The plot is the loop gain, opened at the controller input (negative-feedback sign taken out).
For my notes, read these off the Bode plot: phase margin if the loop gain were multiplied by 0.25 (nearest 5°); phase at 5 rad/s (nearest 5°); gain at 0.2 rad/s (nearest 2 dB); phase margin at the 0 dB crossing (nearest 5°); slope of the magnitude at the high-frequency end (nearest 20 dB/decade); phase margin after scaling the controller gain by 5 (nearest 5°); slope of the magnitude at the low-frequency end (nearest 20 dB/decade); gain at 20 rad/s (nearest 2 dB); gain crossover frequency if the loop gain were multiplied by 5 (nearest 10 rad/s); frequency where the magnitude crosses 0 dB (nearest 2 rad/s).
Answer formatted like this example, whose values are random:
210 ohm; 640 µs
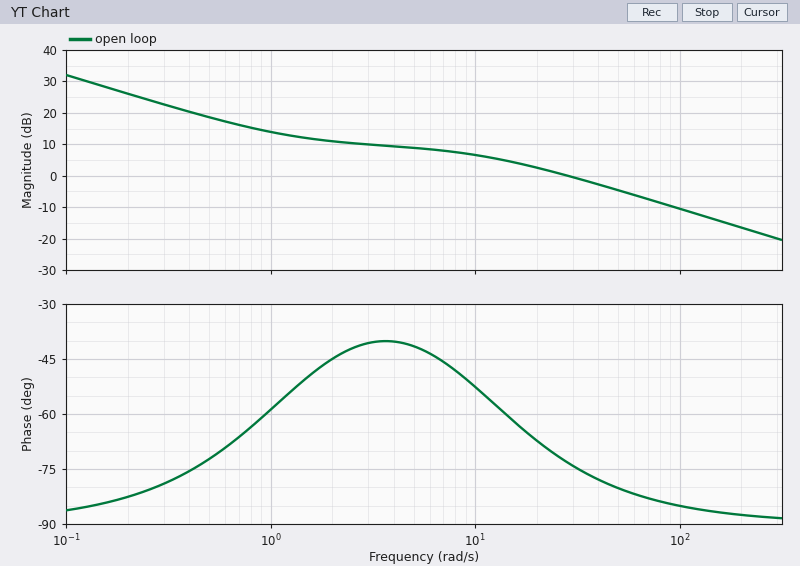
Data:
130°; -40°; 26 dB; 105°; -20 dB/decade; 95°; -20 dB/decade; 2 dB; 150 rad/s; 28 rad/s
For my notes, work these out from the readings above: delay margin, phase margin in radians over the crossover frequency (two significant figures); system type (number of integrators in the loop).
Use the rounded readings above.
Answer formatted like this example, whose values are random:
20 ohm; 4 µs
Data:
0.065 s; 1
